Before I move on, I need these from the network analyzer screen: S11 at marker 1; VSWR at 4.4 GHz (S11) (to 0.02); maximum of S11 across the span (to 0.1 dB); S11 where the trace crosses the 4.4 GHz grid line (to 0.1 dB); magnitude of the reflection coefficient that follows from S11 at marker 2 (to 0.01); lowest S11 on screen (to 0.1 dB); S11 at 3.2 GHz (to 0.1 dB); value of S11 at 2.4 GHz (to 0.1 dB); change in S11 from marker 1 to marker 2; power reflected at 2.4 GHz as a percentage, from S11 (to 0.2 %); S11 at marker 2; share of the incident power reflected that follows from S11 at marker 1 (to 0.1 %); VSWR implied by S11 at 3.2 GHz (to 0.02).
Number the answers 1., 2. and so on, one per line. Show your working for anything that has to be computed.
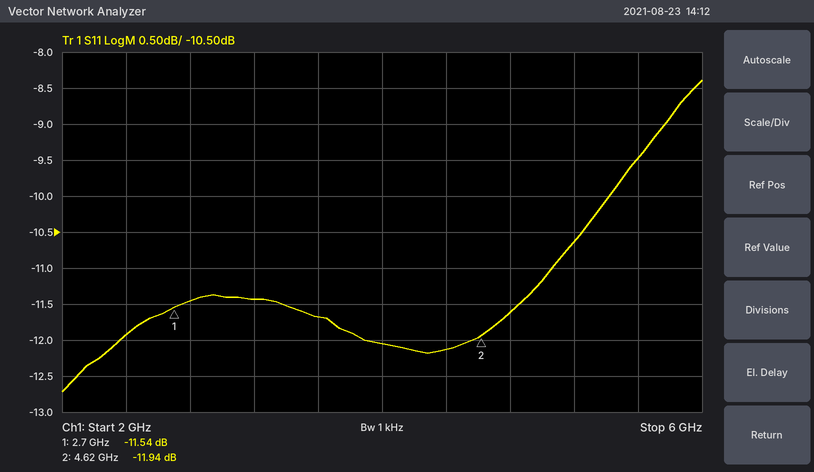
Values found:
1. -11.54 dB
2. |Γ| = 10^(-12.1/20) = 0.2483; VSWR = (1 + 0.2483)/(1 − 0.2483) ≈ 1.66
3. -8.4 dB
4. -12.1 dB
5. 10^(-11.94/20) ≈ 0.25
6. -12.7 dB
7. -11.4 dB
8. -11.9 dB
9. -11.94 − (-11.54) = -0.40 dB
10. 10^(-11.9/10) ≈ 6.46 %, so 6.4 % to the nearest 0.2 %
11. -11.94 dB
12. 10^(-11.54/10) ≈ 7.0 %
13. |Γ| = 10^(-11.4/20) = 0.2692; VSWR = (1 + 0.2692)/(1 − 0.2692) ≈ 1.74
